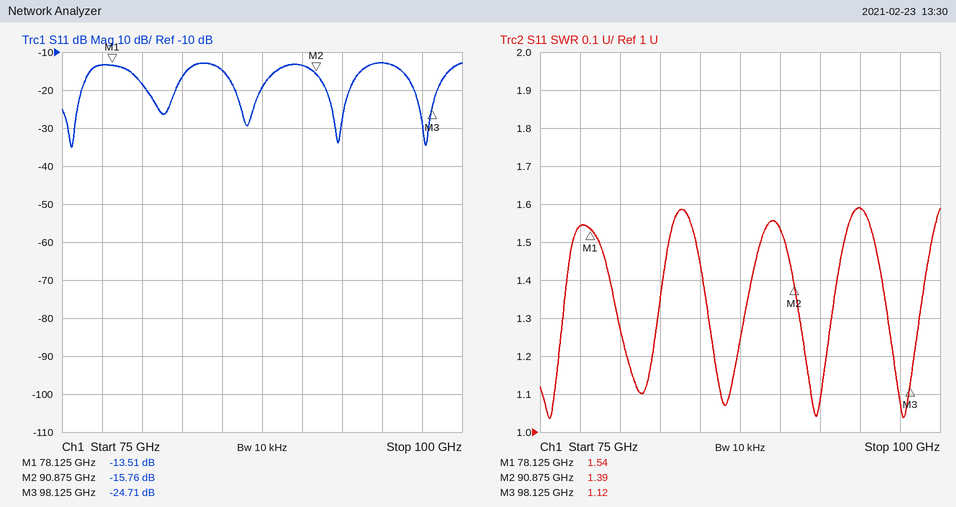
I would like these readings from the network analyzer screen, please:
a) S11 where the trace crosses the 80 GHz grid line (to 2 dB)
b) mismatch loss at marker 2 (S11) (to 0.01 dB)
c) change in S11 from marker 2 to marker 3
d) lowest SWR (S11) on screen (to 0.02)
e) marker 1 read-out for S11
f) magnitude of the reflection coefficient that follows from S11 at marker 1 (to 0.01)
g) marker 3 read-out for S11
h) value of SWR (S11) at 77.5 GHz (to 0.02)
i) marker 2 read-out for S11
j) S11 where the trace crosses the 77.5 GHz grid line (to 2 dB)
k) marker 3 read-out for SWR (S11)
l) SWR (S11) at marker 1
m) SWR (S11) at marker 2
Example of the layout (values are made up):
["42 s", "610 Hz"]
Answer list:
["-18 dB", "0.12 dB", "-8.95 dB", "1.04", "-13.51 dB", "0.21", "-24.71 dB", "1.54", "-15.76 dB", "-14 dB", "1.12", "1.54", "1.39"]
